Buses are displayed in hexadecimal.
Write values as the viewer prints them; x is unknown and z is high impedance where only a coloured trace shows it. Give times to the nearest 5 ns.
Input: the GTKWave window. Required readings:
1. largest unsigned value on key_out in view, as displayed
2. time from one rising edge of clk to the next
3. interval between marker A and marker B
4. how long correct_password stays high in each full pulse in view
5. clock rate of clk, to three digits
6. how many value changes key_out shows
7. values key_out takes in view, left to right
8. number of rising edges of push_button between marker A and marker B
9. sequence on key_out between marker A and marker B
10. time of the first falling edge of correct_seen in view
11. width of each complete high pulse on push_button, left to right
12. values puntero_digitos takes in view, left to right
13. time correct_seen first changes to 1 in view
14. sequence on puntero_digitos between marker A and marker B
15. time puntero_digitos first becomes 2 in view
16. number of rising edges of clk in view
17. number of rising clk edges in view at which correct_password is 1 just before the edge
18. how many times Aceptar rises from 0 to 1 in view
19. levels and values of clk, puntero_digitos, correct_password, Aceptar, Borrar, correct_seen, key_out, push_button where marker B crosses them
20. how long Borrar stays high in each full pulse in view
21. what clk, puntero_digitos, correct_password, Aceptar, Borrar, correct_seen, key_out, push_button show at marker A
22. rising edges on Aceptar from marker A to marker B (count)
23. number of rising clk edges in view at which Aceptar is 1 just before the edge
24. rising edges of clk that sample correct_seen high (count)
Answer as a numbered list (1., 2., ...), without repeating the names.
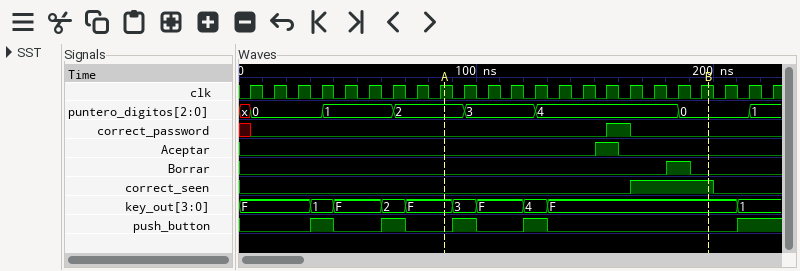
1. F
2. 10 ns
3. 110 ns
4. 10 ns
5. 100 MHz
6. 9
7. F, 1, F, 2, F, 3, F, 4, F, 1
8. 2
9. F, 3, F, 4, F
10. 200 ns
11. 10 ns, 10 ns, 10 ns, 10 ns
12. x, 0, 1, 2, 3, 4, 0, 1
13. 165 ns
14. 2, 3, 4, 0
15. 65 ns
16. 23
17. 1
18. 1
19. clk=1, puntero_digitos=0, correct_password=0, Aceptar=0, Borrar=0, correct_seen=1, key_out=F, push_button=0
20. 10 ns
21. clk=1, puntero_digitos=2, correct_password=0, Aceptar=0, Borrar=0, correct_seen=0, key_out=F, push_button=0
22. 1
23. 1
24. 3
